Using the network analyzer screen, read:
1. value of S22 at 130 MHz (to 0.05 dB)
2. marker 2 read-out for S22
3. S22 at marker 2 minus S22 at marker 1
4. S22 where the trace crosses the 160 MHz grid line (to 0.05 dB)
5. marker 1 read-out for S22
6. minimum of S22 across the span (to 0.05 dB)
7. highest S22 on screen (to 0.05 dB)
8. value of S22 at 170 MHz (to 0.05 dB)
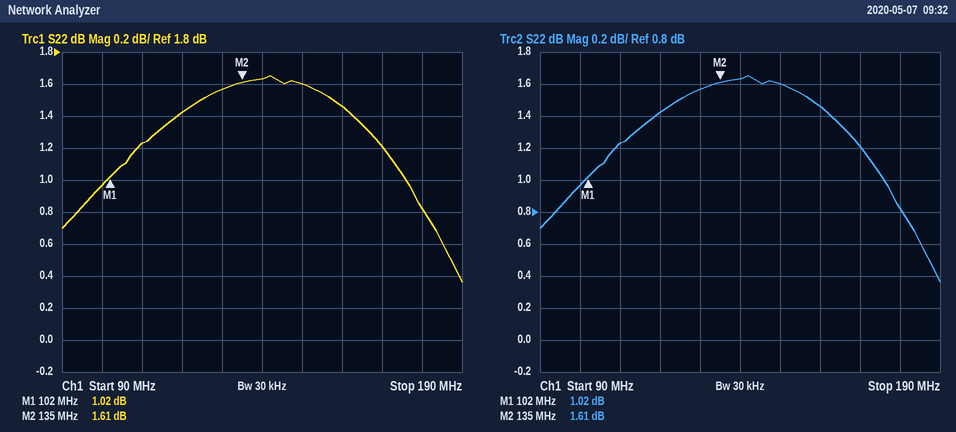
1.55 dB
1.61 dB
0.59 dB
1.45 dB
1.02 dB
0.35 dB
1.65 dB
1.20 dB
